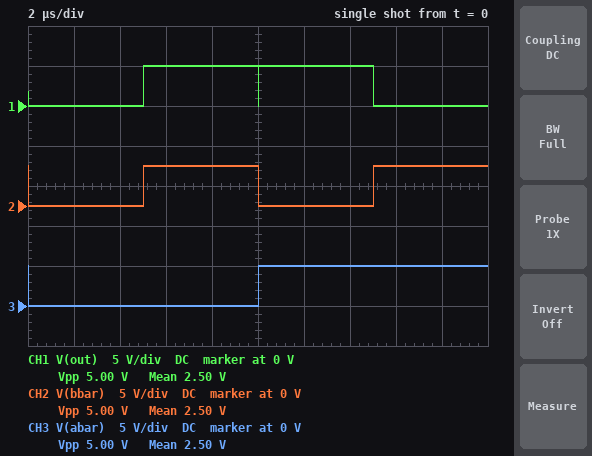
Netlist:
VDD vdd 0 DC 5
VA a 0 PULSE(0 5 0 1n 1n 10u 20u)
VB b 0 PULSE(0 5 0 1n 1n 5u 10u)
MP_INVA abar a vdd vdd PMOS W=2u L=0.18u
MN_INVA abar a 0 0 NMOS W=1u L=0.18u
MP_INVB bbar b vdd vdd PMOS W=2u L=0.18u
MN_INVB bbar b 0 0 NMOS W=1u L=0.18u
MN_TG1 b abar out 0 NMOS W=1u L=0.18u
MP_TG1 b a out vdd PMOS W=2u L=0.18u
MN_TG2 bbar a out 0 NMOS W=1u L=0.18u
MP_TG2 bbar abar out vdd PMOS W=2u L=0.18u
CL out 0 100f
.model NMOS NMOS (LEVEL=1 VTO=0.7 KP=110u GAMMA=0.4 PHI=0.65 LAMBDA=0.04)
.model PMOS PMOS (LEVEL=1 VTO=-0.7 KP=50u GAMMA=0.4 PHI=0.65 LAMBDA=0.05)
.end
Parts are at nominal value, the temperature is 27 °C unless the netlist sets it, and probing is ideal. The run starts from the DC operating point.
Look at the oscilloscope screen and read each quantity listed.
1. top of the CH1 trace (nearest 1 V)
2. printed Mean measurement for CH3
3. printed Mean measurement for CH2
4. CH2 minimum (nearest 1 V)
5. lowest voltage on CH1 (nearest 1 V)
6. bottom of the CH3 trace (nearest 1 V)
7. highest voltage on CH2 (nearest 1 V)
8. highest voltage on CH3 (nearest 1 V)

5 V
2.50 V
2.50 V
0 V
0 V
0 V
5 V
5 V
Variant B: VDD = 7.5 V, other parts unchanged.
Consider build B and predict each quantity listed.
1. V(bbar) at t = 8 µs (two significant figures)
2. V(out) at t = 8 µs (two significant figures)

7.3 V
7.1 V
